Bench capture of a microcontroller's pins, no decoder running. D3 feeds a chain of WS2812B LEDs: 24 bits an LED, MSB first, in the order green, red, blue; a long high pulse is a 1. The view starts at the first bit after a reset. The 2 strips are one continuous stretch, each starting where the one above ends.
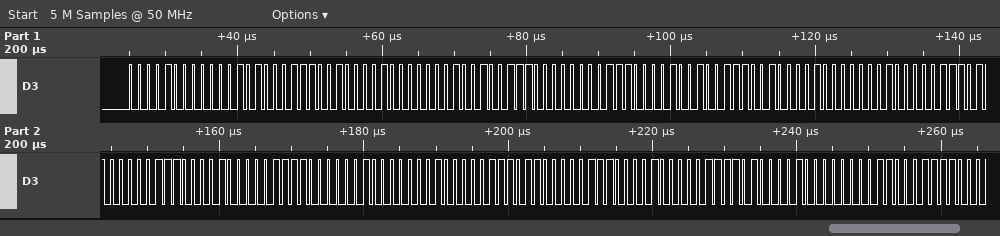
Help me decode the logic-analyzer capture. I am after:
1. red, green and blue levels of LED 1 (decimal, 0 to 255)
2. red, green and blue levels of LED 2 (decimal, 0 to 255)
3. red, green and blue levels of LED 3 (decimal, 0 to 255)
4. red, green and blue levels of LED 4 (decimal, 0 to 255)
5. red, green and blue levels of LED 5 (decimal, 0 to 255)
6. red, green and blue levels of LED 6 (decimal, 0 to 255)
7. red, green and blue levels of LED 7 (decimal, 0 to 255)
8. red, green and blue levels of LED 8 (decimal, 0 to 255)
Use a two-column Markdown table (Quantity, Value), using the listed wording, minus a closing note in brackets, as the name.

| Quantity | Value |
|---|---|
| red, green and blue levels of LED 1 | 10, 8, 57 |
| red, green and blue levels of LED 2 | 9, 8, 56 |
| red, green and blue levels of LED 3 | 9, 7, 57 |
| red, green and blue levels of LED 4 | 8, 8, 58 |
| red, green and blue levels of LED 5 | 8, 7, 60 |
| red, green and blue levels of LED 6 | 8, 8, 59 |
| red, green and blue levels of LED 7 | 8, 7, 61 |
| red, green and blue levels of LED 8 | 6, 8, 60 |
